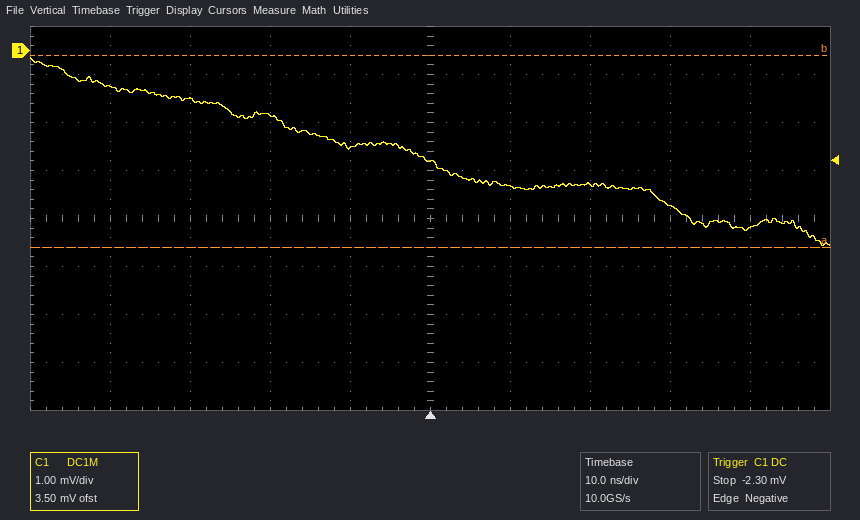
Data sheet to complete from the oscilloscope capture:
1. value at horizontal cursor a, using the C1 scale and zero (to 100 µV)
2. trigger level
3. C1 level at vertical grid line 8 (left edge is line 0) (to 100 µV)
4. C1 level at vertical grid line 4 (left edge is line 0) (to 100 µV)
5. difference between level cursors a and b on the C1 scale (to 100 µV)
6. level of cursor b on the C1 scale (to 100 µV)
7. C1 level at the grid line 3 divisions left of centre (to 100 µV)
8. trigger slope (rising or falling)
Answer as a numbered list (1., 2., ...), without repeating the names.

1. -4.1 mV
2. -2.30 mV
3. -3.2 mV
4. -2.0 mV
5. 4.0 mV
6. -100 µV
7. -1.0 mV
8. falling
